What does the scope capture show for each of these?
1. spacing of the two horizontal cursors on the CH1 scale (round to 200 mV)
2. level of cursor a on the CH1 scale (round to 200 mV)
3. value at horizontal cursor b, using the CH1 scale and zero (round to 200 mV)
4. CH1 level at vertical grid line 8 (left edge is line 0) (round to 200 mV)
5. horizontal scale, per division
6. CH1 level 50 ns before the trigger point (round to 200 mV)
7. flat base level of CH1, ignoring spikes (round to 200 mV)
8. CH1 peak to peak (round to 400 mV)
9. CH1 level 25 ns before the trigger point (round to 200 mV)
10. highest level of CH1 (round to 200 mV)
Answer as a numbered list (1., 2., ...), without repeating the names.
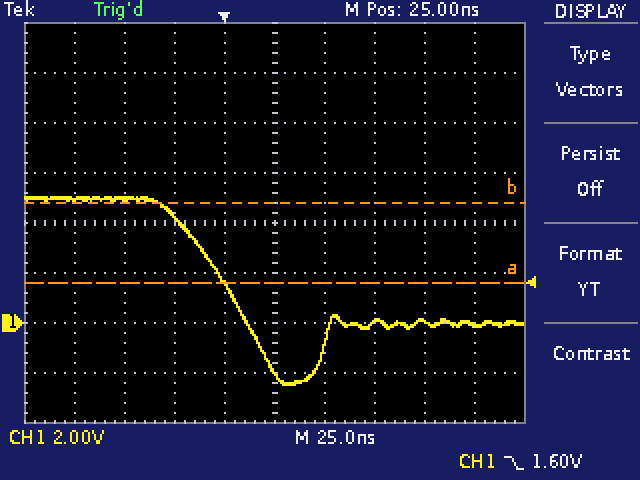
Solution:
1. 3.2 V
2. 1.6 V
3. 4.8 V
4. 0.0 V
5. 25 ns
6. 5.0 V
7. 0.0 V
8. 7.6 V
9. 4.2 V
10. 5.0 V
